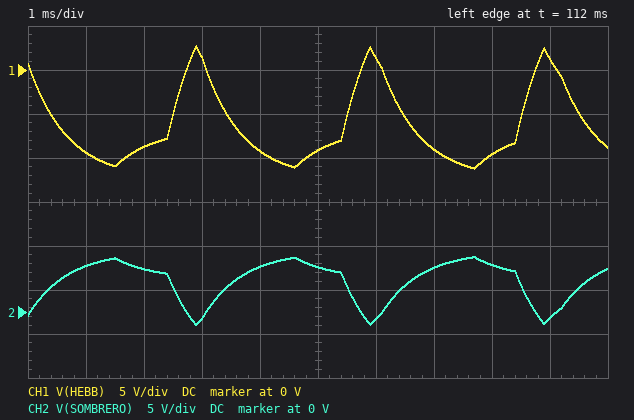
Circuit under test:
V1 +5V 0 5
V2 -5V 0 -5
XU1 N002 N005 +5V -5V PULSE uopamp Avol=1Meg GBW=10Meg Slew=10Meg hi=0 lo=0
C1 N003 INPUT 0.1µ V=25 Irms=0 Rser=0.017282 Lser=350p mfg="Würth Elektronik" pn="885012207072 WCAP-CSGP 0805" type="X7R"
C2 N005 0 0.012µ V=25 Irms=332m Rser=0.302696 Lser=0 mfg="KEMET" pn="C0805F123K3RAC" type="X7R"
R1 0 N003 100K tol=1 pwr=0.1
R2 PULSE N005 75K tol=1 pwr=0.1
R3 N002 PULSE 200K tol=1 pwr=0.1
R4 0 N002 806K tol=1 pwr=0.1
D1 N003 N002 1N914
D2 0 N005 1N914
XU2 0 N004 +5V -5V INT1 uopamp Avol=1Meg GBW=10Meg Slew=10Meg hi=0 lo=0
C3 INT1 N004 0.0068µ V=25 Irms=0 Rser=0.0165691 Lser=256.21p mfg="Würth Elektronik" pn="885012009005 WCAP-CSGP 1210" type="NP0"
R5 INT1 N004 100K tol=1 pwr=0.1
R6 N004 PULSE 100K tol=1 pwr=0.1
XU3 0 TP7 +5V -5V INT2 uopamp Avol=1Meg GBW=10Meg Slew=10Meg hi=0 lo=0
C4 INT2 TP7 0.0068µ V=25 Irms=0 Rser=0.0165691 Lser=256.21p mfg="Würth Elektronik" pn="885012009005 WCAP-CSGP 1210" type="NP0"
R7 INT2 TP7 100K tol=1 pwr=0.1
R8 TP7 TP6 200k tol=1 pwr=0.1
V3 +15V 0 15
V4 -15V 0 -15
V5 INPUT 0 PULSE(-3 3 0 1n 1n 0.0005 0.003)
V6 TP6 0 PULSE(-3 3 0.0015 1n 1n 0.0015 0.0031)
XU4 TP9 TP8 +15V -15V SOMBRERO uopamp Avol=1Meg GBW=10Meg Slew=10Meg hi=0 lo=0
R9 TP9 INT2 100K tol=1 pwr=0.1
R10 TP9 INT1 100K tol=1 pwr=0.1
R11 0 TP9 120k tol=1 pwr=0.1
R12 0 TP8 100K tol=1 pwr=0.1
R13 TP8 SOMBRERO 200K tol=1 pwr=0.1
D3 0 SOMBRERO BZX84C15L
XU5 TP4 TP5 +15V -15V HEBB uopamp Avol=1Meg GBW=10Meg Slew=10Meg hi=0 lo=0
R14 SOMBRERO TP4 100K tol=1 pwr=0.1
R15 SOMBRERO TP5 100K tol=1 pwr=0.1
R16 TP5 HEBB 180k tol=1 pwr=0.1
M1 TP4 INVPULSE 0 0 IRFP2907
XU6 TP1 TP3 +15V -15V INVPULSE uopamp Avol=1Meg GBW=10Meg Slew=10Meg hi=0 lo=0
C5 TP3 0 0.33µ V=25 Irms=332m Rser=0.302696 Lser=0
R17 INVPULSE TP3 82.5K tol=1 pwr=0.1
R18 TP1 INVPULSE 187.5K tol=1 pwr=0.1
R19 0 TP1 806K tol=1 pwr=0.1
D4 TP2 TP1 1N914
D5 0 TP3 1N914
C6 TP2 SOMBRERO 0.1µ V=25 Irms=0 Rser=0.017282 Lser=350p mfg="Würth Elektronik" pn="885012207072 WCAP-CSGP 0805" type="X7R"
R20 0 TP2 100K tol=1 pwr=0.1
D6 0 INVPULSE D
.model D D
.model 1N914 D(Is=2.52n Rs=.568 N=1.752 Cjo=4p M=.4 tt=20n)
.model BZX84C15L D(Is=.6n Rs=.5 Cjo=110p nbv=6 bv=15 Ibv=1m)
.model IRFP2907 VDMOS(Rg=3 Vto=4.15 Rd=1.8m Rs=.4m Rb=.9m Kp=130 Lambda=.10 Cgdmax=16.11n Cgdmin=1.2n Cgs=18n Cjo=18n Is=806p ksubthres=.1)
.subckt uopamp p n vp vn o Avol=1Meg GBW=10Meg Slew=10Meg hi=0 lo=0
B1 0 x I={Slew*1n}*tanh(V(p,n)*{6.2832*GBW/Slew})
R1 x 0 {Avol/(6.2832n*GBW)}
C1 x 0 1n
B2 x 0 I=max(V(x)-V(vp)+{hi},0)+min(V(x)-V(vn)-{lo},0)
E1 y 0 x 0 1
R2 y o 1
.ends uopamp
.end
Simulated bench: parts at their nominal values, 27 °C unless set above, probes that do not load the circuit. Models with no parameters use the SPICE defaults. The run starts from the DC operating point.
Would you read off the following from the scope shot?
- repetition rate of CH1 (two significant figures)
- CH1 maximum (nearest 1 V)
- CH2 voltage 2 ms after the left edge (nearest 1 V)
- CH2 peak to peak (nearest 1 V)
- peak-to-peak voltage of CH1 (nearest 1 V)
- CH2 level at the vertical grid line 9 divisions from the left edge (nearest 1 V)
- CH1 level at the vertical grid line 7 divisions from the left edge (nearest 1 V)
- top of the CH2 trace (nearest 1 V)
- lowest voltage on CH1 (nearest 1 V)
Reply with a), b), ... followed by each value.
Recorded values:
a) 330 Hz
b) 3 V
c) 5 V
d) 8 V
e) 14 V
f) -1 V
g) -9 V
h) 6 V
i) -11 V
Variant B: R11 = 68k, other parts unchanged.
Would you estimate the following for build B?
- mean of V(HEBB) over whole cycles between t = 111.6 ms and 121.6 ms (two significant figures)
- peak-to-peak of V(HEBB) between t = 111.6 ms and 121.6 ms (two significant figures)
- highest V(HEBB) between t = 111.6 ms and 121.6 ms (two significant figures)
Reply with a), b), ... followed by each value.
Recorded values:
a) -5.3 V
b) 11 V
c) 2.2 V
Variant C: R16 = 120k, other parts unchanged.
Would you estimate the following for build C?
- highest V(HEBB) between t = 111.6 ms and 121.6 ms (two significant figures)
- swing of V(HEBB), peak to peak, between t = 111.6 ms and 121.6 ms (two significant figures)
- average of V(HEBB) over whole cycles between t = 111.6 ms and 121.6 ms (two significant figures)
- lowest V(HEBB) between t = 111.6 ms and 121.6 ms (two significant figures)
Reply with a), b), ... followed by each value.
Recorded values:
a) 1.8 V
b) 9.3 V
c) -4.3 V
d) -7.5 V
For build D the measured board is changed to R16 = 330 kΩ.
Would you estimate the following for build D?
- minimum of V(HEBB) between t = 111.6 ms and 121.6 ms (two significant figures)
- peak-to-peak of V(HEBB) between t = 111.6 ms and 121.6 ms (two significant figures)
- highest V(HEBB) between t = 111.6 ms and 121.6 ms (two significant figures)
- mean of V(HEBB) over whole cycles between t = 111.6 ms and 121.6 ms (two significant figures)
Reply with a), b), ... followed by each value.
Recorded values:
a) -15 V
b) 20 V
c) 5.0 V
d) -11 V
